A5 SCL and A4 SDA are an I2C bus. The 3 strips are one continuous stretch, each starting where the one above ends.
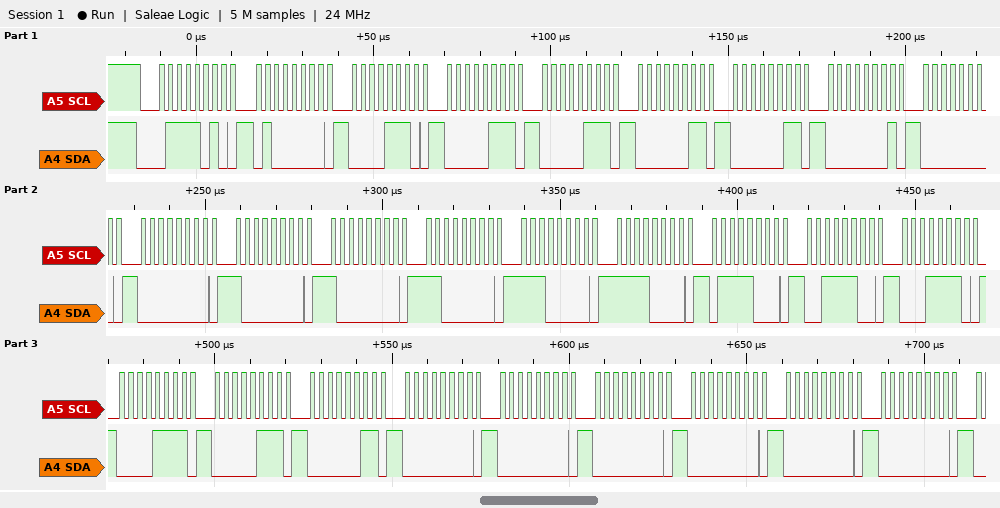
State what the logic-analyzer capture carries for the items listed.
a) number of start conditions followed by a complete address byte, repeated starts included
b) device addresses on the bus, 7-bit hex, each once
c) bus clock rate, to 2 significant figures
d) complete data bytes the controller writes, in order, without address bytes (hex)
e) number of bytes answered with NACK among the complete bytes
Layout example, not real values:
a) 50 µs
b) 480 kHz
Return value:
a) 1
b) 0x3D
c) 400 kHz
d) 40 0E 07 07 03 03 01 00 00 80 80 C0 E0 F0 78 3C 1E 0F 07 03 00 00 00 00 00 00
e) 0
